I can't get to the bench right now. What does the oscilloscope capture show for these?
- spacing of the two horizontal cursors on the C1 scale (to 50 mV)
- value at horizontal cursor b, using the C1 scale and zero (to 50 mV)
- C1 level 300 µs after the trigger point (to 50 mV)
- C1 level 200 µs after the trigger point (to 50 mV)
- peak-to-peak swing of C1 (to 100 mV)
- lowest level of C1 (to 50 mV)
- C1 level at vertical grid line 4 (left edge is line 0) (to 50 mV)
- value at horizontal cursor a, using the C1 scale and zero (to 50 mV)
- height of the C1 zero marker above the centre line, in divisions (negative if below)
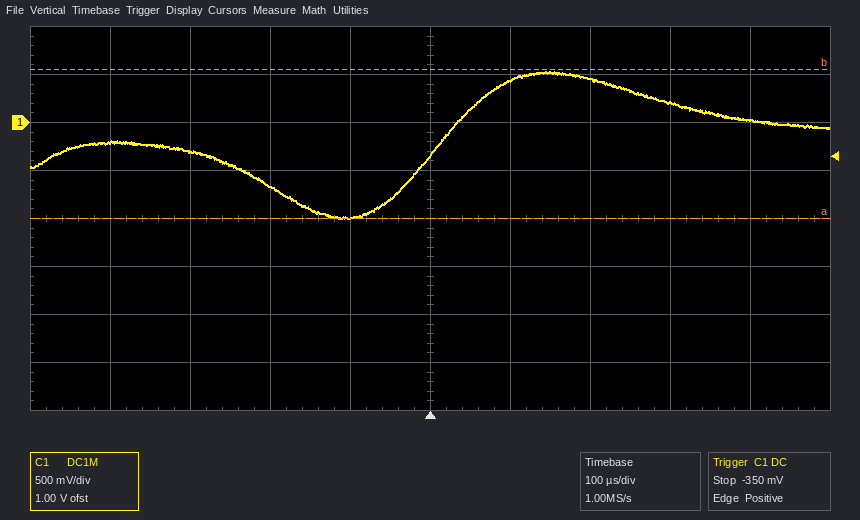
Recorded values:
1.55 V
550 mV
200 mV
450 mV
1.50 V
-1.00 V
-1.00 V
-1.00 V
+2.0 div
